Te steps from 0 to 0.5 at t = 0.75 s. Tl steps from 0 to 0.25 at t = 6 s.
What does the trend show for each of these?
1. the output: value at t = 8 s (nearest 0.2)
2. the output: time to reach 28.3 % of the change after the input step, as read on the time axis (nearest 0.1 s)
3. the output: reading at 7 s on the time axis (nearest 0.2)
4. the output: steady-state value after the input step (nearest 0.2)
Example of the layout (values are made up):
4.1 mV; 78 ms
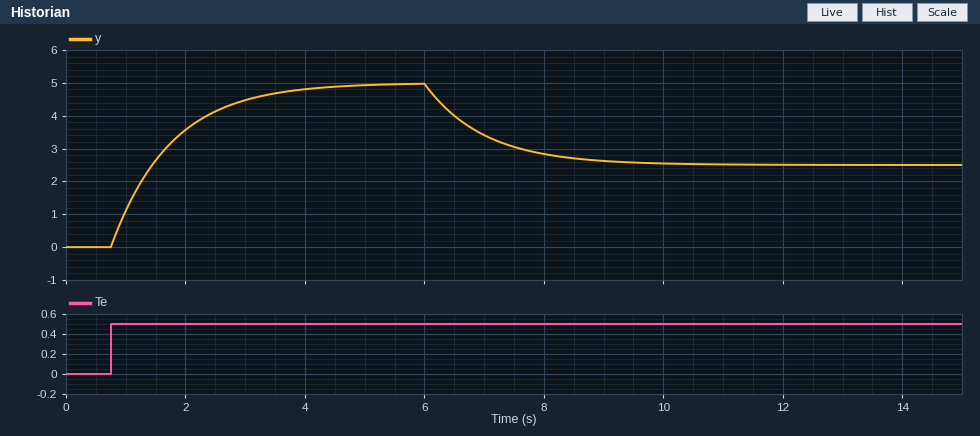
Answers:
2.8; 1.1 s; 3.4; 5.0
